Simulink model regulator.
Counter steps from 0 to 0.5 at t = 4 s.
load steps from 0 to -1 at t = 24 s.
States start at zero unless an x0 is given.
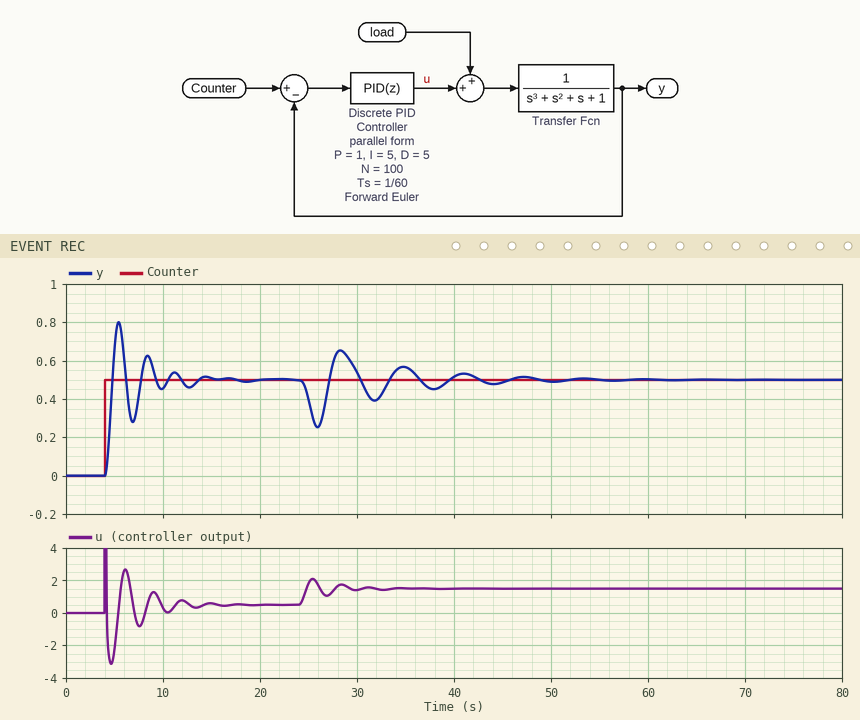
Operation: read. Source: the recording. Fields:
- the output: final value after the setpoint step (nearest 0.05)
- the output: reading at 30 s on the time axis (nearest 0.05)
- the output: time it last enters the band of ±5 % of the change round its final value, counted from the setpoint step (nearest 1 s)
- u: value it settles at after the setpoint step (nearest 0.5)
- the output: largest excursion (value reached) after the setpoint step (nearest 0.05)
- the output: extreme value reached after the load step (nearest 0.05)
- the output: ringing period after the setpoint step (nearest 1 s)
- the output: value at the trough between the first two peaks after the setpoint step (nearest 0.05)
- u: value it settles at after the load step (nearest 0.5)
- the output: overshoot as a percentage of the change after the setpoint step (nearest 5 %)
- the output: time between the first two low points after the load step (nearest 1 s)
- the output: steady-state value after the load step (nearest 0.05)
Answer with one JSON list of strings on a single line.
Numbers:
["0.50", "0.55", "9 s", "0.5", "0.80", "0.25", "3 s", "0.30", "1.5", "60 %", "6 s", "0.50"]
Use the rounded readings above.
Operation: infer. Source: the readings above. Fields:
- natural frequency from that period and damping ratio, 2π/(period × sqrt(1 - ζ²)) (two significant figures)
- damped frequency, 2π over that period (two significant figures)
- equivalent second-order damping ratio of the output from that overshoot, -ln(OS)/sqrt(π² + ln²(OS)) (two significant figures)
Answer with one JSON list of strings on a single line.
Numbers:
["2.1 rad/s", "2.1 rad/s", "0.16"]
